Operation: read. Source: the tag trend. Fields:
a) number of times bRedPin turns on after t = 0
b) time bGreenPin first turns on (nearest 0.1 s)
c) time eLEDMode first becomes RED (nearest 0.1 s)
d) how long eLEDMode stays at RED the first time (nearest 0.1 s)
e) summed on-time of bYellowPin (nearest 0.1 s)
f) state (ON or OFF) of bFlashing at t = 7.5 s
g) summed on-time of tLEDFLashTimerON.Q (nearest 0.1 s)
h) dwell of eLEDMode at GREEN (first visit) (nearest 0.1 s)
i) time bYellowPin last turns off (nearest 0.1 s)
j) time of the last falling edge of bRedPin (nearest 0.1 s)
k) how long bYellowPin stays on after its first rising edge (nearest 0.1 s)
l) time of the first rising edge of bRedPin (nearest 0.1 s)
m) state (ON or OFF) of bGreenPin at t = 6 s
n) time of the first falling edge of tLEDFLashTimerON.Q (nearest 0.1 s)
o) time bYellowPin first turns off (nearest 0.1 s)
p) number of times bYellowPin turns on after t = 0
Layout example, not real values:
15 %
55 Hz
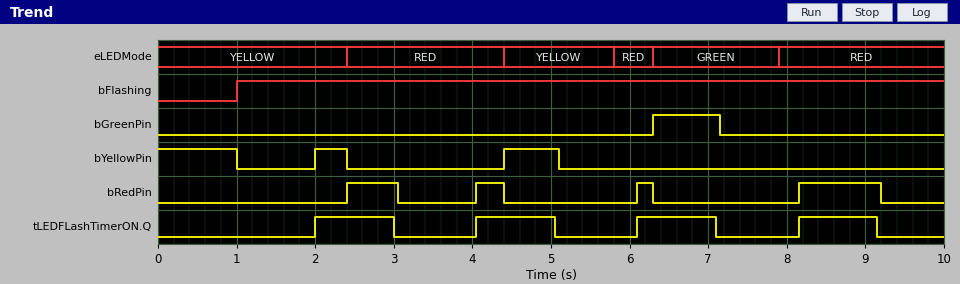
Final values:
4
6.3 s
2.4 s
2.0 s
2.1 s
ON
4.0 s
1.6 s
5.1 s
9.2 s
0.4 s
2.4 s
OFF
3.0 s
1.0 s
2
